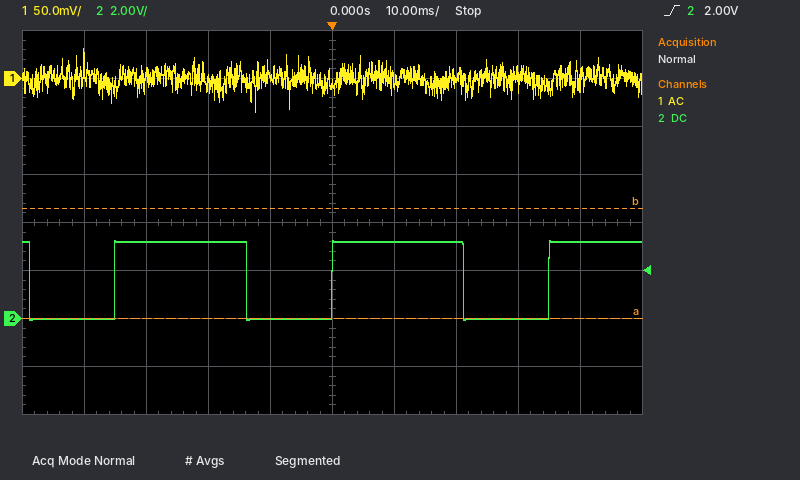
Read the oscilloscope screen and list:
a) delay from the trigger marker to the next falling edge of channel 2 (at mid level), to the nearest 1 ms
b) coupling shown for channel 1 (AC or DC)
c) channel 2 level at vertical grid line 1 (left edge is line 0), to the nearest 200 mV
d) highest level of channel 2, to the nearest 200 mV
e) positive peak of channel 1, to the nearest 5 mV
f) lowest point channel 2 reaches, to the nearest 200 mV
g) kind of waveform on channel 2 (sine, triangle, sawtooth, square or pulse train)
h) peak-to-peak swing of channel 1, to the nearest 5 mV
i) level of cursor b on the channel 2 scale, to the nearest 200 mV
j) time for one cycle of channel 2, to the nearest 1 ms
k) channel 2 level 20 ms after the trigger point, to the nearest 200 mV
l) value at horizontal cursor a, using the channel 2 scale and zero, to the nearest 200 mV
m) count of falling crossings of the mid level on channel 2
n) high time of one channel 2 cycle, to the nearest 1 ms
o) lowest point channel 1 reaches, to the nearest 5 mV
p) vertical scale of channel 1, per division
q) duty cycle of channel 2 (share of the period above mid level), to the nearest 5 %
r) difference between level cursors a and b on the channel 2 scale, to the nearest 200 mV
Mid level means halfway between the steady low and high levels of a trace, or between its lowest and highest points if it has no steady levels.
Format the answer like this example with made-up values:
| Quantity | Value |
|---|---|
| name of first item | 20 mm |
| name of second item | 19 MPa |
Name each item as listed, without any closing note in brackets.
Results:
| Quantity | Value |
|---|---|
| delay from the trigger marker to the next falling edge of channel 2 (at mid level), to the nearest 1 ms | 21 ms |
| coupling shown for channel 1 | AC |
| channel 2 level at vertical grid line 1 (left edge is line 0), to the nearest 200 mV | 0.0 V |
| highest level of channel 2, to the nearest 200 mV | 3.2 V |
| positive peak of channel 1, to the nearest 5 mV | 30 mV |
| lowest point channel 2 reaches, to the nearest 200 mV | 0.0 V |
| kind of waveform on channel 2 | pulse train |
| peak-to-peak swing of channel 1, to the nearest 5 mV | 65 mV |
| level of cursor b on the channel 2 scale, to the nearest 200 mV | 4.6 V |
| time for one cycle of channel 2, to the nearest 1 ms | 35 ms |
| channel 2 level 20 ms after the trigger point, to the nearest 200 mV | 3.2 V |
| value at horizontal cursor a, using the channel 2 scale and zero, to the nearest 200 mV | 0.0 V |
| count of falling crossings of the mid level on channel 2 | 3 |
| high time of one channel 2 cycle, to the nearest 1 ms | 21 ms |
| lowest point channel 1 reaches, to the nearest 5 mV | -35 mV |
| vertical scale of channel 1, per division | 50 mV |
| duty cycle of channel 2 (share of the period above mid level), to the nearest 5 % | 60 % |
| difference between level cursors a and b on the channel 2 scale, to the nearest 200 mV | 4.6 V |
